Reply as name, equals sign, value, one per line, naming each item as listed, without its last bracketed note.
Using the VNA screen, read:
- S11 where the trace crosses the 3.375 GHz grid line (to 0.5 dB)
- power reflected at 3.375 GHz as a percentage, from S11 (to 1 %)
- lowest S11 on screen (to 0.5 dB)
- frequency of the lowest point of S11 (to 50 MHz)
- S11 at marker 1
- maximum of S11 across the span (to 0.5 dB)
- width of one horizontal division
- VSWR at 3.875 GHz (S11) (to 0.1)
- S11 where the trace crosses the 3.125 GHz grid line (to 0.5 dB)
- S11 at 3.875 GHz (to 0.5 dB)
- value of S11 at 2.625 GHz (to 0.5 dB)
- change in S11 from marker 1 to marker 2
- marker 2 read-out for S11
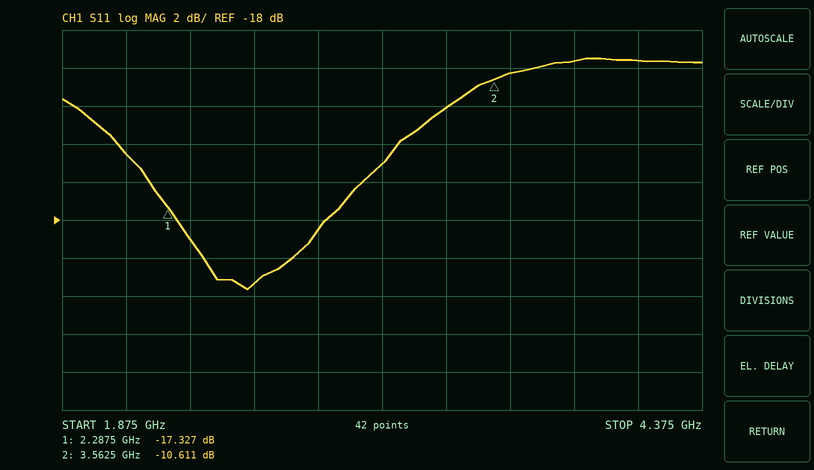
S11 where the trace crosses the 3.375 GHz grid line = -12.0 dB
power reflected at 3.375 GHz as a percentage, from S11 = 6 %
lowest S11 on screen = -21.5 dB
frequency of the lowest point of S11 = 2.60 GHz
S11 at marker 1 = -17.327 dB
maximum of S11 across the span = -9.5 dB
width of one horizontal division = 250 MHz
VSWR at 3.875 GHz (S11) = 2.0
S11 where the trace crosses the 3.125 GHz grid line = -15.0 dB
S11 at 3.875 GHz = -9.5 dB
value of S11 at 2.625 GHz = -21.5 dB
change in S11 from marker 1 to marker 2 = 6.716 dB
marker 2 read-out for S11 = -10.611 dB
